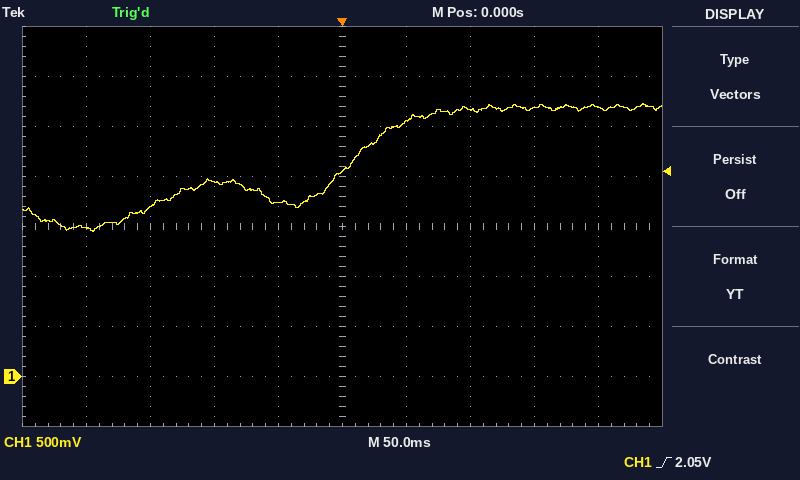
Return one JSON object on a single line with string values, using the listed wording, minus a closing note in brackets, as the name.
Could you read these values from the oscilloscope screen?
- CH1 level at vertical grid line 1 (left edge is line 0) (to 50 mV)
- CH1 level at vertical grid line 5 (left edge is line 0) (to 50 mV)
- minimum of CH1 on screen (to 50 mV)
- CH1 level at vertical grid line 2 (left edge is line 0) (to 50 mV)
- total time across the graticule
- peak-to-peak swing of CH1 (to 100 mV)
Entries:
{"CH1 level at vertical grid line 1 (left edge is line 0)": "1.50 V", "CH1 level at vertical grid line 5 (left edge is line 0)": "2.05 V", "minimum of CH1 on screen": "1.45 V", "CH1 level at vertical grid line 2 (left edge is line 0)": "1.70 V", "total time across the graticule": "500 ms", "peak-to-peak swing of CH1": "1.30 V"}
